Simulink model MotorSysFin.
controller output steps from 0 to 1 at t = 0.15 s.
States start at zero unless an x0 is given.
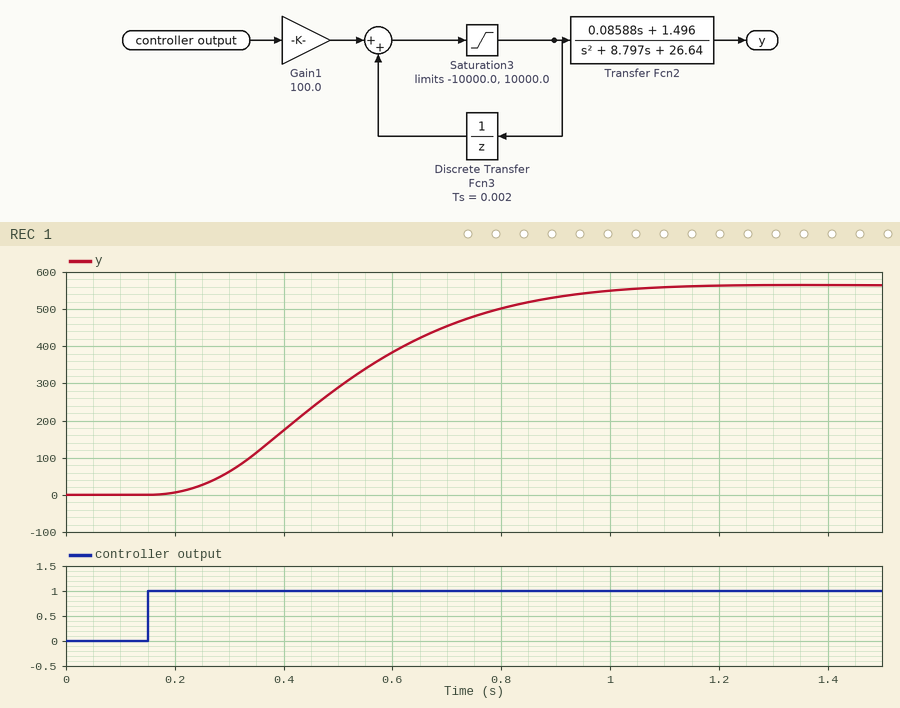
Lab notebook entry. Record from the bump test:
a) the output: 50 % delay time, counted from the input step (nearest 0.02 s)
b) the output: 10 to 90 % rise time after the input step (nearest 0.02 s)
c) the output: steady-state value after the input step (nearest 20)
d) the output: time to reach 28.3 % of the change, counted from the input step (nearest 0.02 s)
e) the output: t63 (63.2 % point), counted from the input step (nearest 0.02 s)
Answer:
0.34 s
0.52 s
560
0.24 s
0.42 s
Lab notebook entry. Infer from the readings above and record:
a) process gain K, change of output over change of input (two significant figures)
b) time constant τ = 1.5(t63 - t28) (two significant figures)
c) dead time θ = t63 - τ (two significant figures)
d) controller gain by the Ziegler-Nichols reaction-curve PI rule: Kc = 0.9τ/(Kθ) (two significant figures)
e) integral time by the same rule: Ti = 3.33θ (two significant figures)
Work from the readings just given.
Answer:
560
0.27 s
0.15 s
0.0029
0.50 s
